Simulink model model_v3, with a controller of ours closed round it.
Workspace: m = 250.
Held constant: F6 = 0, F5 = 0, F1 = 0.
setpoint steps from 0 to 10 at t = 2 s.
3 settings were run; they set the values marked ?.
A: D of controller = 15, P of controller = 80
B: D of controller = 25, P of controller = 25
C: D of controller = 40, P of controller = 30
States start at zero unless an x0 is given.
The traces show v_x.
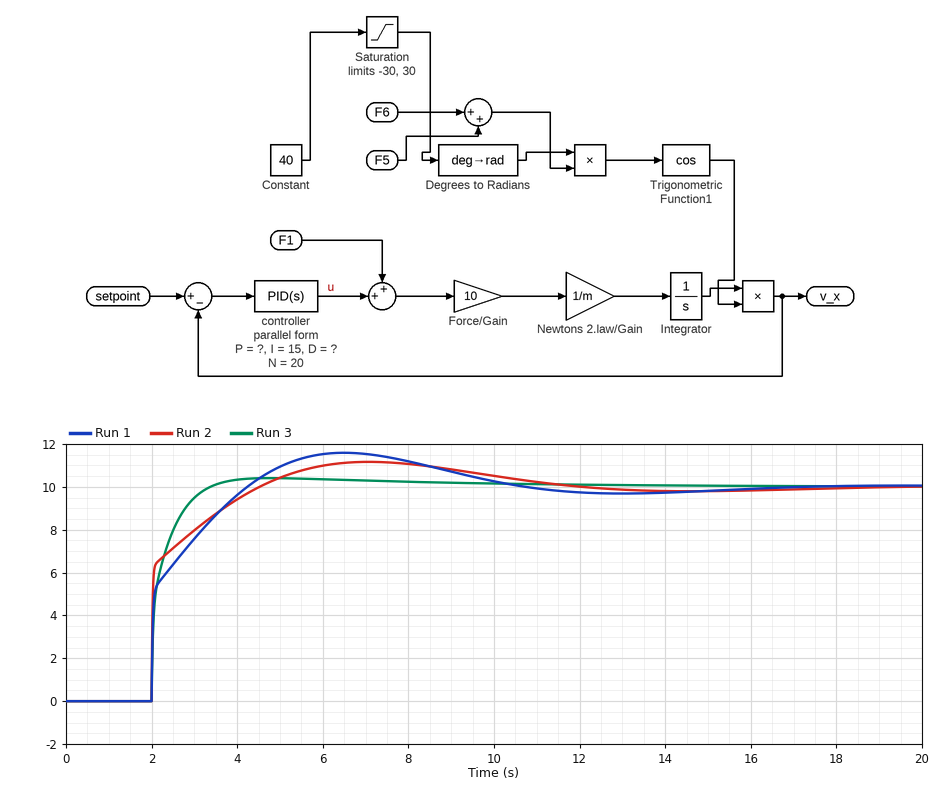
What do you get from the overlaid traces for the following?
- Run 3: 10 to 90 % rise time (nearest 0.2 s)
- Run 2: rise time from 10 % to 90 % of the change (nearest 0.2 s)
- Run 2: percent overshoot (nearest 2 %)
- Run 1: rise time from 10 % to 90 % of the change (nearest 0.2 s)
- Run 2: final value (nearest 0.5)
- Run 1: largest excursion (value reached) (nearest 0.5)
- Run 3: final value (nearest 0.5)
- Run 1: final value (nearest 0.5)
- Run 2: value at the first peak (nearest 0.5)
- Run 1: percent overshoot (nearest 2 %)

0.8 s
1.6 s
12 %
1.6 s
10.0
11.5
10.0
10.0
11.0
16 %
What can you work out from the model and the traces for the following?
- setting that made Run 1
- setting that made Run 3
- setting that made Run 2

B
A
C
